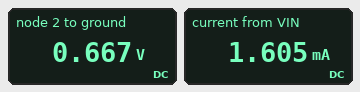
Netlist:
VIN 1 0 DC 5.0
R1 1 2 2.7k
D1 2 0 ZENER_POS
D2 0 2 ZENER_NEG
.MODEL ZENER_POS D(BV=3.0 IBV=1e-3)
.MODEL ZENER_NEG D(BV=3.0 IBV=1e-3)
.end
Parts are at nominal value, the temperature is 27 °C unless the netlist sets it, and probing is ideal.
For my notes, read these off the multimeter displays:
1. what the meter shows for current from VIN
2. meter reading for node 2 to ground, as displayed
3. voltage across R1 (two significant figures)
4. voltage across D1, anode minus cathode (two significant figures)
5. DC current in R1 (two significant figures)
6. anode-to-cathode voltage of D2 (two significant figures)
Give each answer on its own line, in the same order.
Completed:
1.605 mA
0.667 V
4.3 V
670 mV
1.6 mA
-670 mV
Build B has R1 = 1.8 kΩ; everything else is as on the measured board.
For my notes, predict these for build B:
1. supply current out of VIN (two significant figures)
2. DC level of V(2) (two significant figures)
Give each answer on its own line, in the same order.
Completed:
2.4 mA
680 mV
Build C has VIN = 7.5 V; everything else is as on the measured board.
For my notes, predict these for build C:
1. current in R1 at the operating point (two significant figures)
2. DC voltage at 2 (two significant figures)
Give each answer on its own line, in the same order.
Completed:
2.5 mA
680 mV
